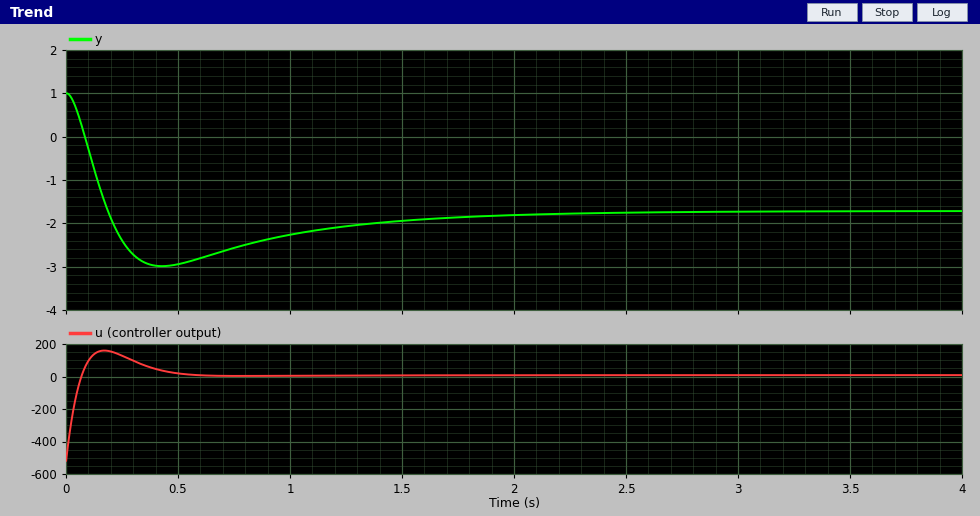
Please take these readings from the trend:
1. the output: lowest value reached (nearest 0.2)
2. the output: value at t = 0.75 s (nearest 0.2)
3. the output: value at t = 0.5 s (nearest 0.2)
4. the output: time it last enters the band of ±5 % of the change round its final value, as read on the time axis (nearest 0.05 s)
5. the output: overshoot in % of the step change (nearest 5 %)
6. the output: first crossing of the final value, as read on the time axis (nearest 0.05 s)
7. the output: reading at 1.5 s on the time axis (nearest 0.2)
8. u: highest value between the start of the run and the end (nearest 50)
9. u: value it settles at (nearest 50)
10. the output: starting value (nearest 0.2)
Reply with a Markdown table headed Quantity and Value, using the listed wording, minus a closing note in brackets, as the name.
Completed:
| Quantity | Value |
|---|---|
| the output: lowest value reached | -3.0 |
| the output: value at t = 0.75 s | -2.6 |
| the output: value at t = 0.5 s | -3.0 |
| the output: time it last enters the band of ±5 % of the change round its final value, as read on the time axis | 1.80 s |
| the output: overshoot in % of the step change | 45 % |
| the output: first crossing of the final value, as read on the time axis | 0.20 s |
| the output: reading at 1.5 s on the time axis | -2.0 |
| u: highest value between the start of the run and the end | 150 |
| u: value it settles at | 0 |
| the output: starting value | 1.0 |
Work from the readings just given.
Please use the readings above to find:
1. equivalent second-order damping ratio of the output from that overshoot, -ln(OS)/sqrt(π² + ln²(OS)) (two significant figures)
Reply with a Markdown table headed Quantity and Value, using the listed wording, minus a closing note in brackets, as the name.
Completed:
| Quantity | Value |
|---|---|
| equivalent second-order damping ratio of the output from that overshoot, -ln(OS)/sqrt(π² + ln²(OS)) | 0.25 |
